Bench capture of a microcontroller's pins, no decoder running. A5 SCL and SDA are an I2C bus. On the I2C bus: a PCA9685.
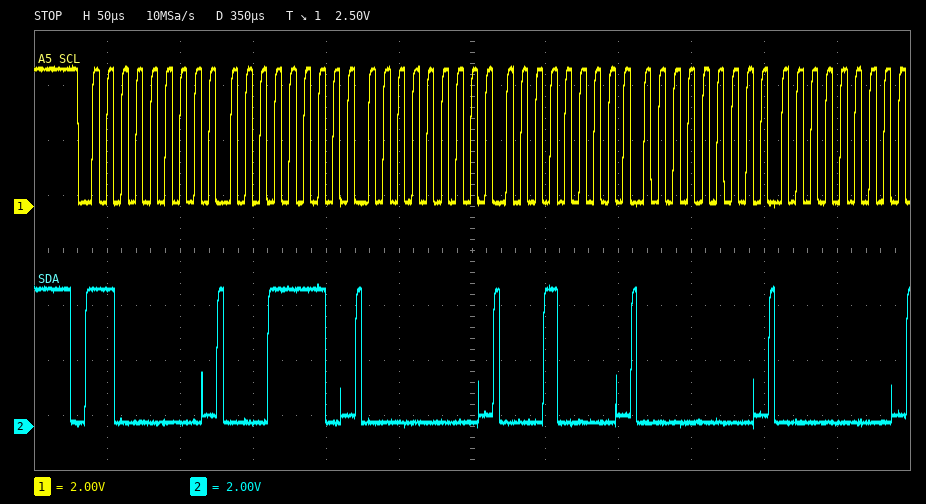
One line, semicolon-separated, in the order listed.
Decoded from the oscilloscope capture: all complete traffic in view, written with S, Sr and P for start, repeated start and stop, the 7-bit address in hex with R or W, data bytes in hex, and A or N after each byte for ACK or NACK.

S 60W A 1E A 00 A 10 A 00 A 00 A
